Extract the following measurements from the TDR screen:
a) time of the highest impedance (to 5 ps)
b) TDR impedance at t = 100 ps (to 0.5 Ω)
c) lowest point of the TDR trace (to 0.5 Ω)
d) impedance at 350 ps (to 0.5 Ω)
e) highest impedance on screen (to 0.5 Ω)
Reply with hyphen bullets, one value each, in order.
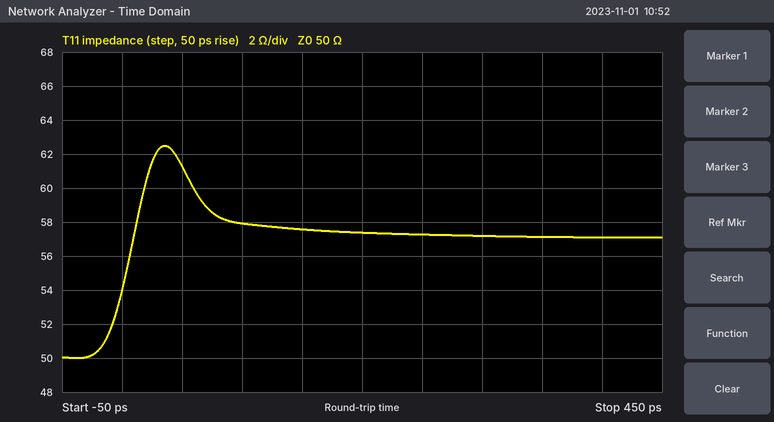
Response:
- 35 ps
- 58.0 Ω
- 50.0 Ω
- 57.0 Ω
- 62.5 Ω
